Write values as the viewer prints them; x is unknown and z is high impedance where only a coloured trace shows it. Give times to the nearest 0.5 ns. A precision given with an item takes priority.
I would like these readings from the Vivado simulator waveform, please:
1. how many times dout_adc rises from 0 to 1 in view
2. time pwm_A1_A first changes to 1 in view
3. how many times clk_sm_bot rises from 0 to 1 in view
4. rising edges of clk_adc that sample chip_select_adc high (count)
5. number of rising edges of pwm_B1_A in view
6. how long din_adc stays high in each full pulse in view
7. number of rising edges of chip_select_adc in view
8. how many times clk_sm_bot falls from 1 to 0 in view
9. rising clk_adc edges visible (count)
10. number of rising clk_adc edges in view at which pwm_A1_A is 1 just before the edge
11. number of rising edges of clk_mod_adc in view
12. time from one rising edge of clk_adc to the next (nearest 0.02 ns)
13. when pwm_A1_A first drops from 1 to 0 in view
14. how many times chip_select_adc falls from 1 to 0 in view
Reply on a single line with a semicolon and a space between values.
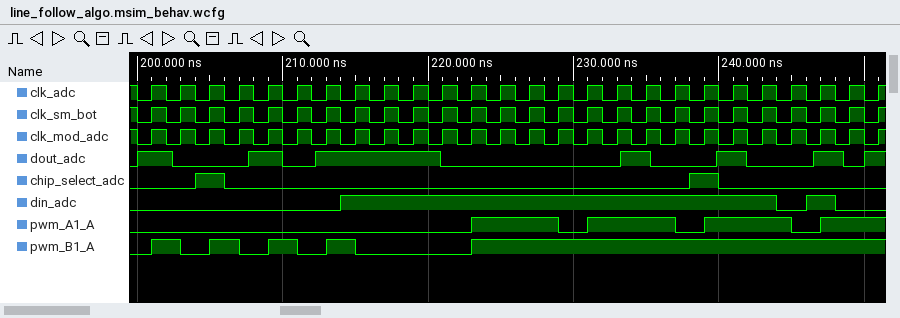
7; 223 ns; 26; 2; 5; 30 ns, 2 ns; 2; 26; 26; 11; 26; 2 ns; 229 ns; 2
